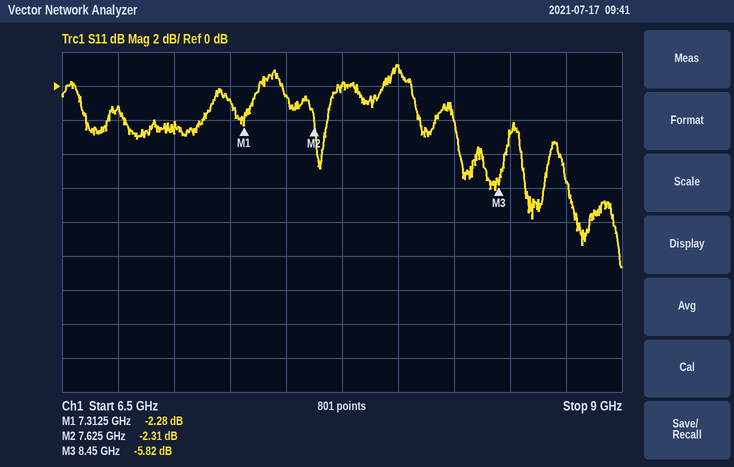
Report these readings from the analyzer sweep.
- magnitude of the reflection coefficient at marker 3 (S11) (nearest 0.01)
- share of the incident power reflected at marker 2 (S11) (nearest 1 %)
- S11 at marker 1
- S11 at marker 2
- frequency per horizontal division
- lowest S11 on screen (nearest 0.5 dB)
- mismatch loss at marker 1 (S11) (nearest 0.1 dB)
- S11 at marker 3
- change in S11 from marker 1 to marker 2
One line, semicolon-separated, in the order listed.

0.51; 59 %; -2.28 dB; -2.31 dB; 250 MHz; -10.5 dB; 3.9 dB; -5.82 dB; -0.03 dB
